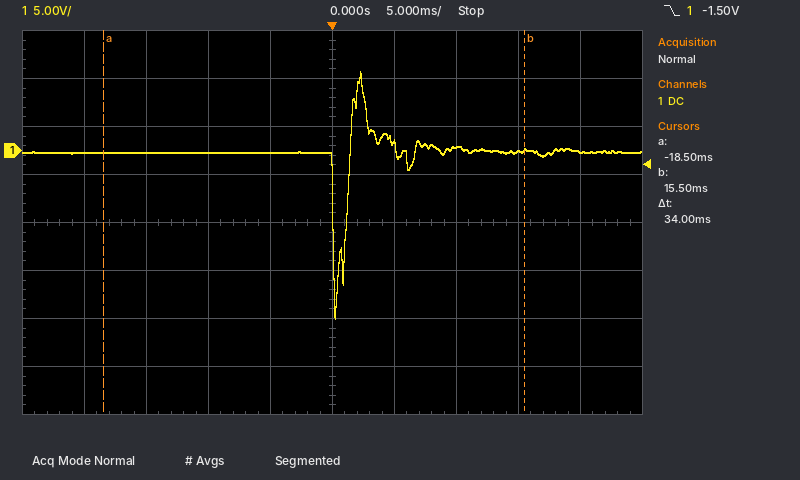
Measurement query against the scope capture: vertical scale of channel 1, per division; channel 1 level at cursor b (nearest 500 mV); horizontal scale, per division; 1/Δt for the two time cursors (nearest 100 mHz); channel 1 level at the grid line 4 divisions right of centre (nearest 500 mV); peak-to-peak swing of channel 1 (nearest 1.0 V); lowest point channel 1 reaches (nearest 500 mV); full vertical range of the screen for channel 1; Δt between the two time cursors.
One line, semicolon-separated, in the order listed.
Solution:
5 V; 0.0 V; 5 ms; 29.4 Hz; 0.0 V; 26.0 V; -17.5 V; 40 V; 34 ms
